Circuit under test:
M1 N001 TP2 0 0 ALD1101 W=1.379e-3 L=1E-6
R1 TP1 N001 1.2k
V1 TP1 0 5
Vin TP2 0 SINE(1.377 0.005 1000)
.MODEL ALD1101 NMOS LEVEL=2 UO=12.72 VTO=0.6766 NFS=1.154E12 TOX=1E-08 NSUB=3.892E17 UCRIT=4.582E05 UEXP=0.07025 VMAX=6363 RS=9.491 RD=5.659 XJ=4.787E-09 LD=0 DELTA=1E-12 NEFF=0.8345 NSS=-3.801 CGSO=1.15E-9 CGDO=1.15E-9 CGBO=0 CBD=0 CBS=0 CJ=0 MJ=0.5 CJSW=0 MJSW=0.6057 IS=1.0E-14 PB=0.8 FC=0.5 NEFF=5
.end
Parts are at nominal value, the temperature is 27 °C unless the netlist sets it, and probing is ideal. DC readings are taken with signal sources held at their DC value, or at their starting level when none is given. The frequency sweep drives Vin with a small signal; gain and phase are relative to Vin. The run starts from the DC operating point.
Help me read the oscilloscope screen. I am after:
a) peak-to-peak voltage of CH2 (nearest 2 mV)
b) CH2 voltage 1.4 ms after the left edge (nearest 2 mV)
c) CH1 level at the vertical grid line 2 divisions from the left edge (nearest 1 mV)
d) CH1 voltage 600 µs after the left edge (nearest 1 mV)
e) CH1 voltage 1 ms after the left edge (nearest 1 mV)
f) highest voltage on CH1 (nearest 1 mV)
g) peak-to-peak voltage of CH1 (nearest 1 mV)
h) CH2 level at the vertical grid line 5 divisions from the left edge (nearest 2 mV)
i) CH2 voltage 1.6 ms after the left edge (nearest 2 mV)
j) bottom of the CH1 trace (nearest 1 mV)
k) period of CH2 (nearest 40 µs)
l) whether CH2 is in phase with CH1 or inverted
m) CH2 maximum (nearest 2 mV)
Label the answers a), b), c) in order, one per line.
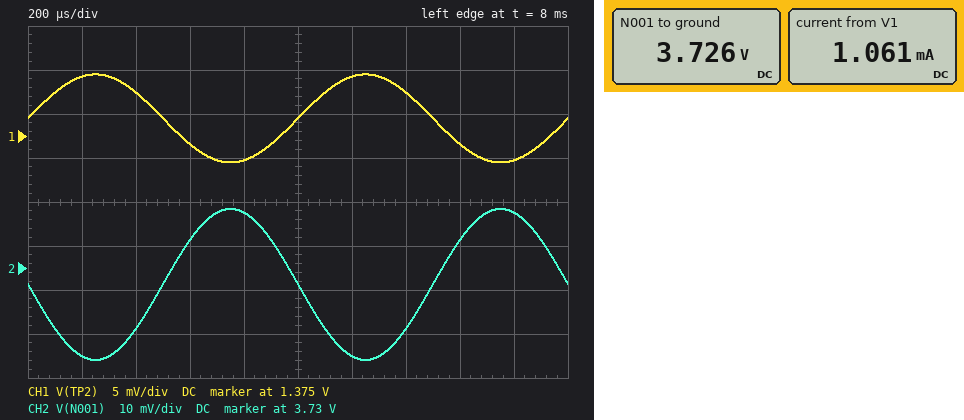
a) 34 mV
b) 3.716 V
c) 1.380 V
d) 1.374 V
e) 1.377 V
f) 1.382 V
g) 10 mV
h) 3.726 V
i) 3.736 V
j) 1.372 V
k) 1.00 ms
l) inverted
m) 3.744 V
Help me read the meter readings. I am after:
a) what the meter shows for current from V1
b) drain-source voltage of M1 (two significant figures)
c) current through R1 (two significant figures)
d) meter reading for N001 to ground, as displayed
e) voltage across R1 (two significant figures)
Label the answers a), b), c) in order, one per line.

a) 1.061 mA
b) 3.7 V
c) 1.1 mA
d) 3.726 V
e) 1.3 V
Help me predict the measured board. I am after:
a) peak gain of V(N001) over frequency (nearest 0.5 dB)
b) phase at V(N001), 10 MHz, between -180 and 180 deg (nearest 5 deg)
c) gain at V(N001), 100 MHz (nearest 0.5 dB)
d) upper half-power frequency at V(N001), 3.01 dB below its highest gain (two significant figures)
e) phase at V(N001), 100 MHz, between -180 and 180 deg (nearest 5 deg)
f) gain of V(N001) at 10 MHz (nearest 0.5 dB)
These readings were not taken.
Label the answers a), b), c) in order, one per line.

a) 10.5 dB
b) 170 deg
c) 7.5 dB
d) 95 MHz
e) 110 deg
f) 10.5 dB
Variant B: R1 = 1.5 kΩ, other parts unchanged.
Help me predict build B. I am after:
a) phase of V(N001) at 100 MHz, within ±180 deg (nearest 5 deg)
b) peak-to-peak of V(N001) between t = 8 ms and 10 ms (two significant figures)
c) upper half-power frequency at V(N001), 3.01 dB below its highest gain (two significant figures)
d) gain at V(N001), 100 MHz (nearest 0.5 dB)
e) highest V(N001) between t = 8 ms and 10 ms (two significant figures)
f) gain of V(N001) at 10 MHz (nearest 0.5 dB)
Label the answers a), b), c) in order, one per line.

a) 105 deg
b) 43 mV
c) 73 MHz
d) 8.0 dB
e) 3.4 V
f) 12.5 dB
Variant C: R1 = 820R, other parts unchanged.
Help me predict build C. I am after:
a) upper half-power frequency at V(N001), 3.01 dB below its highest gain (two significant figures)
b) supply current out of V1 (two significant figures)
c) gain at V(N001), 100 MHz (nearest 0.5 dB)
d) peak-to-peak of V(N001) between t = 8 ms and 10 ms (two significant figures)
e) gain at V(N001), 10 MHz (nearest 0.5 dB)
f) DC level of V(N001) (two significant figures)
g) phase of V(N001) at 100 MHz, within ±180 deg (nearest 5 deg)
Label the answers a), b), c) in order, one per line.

a) 160 MHz
b) 1.1 mA
c) 6.0 dB
d) 24 mV
e) 7.5 dB
f) 4.1 V
g) 120 deg
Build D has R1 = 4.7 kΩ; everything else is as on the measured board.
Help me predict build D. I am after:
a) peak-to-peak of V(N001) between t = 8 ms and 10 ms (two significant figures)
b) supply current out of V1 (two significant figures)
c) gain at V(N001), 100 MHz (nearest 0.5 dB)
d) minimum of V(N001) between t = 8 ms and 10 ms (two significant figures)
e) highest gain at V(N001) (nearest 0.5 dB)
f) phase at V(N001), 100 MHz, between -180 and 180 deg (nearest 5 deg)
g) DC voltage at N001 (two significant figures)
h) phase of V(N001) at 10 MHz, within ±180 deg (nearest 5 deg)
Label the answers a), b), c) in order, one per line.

a) 26 mV
b) 980 µA
c) 3.5 dB
d) 400 mV
e) 6.0 dB
f) 90 deg
g) 410 mV
h) 170 deg
